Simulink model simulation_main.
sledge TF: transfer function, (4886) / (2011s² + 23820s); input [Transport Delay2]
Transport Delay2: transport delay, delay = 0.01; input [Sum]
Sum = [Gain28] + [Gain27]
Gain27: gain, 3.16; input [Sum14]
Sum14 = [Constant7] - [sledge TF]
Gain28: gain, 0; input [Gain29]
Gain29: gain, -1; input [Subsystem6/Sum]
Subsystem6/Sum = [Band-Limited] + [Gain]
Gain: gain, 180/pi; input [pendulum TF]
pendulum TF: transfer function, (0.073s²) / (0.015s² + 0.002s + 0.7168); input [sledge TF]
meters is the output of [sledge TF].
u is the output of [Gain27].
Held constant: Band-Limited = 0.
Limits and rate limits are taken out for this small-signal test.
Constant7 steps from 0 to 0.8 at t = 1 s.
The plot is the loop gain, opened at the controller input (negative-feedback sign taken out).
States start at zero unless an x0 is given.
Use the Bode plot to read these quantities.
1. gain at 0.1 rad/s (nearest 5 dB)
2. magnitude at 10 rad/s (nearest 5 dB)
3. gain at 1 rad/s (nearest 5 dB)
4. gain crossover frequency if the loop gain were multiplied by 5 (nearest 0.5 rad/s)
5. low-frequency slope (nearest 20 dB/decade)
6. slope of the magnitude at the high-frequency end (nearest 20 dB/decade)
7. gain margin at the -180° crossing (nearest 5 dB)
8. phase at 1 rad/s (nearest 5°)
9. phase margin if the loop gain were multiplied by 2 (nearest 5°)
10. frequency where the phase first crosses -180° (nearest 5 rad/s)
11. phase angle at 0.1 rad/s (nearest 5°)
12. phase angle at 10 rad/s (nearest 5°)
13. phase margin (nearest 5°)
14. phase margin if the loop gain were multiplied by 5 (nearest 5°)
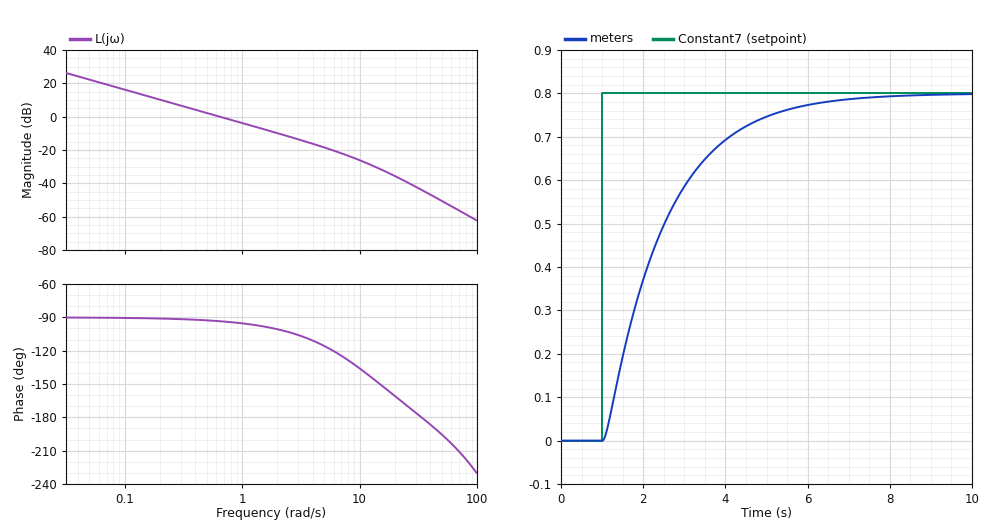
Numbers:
15 dB
-25 dB
-5 dB
3.0 rad/s
-20 dB/decade
-40 dB/decade
45 dB
-95°
85°
35 rad/s
-90°
-135°
85°
75°
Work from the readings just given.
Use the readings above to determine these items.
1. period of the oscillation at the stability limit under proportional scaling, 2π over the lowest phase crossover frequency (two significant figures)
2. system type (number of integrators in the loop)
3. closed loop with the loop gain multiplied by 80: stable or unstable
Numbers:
0.18 s
1
stable
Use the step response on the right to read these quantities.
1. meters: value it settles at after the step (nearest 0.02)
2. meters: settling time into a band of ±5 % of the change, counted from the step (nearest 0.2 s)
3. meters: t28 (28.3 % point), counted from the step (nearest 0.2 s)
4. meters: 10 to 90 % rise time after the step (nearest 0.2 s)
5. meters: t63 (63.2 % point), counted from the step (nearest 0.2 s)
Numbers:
0.80
4.4 s
0.6 s
3.2 s
1.6 s
